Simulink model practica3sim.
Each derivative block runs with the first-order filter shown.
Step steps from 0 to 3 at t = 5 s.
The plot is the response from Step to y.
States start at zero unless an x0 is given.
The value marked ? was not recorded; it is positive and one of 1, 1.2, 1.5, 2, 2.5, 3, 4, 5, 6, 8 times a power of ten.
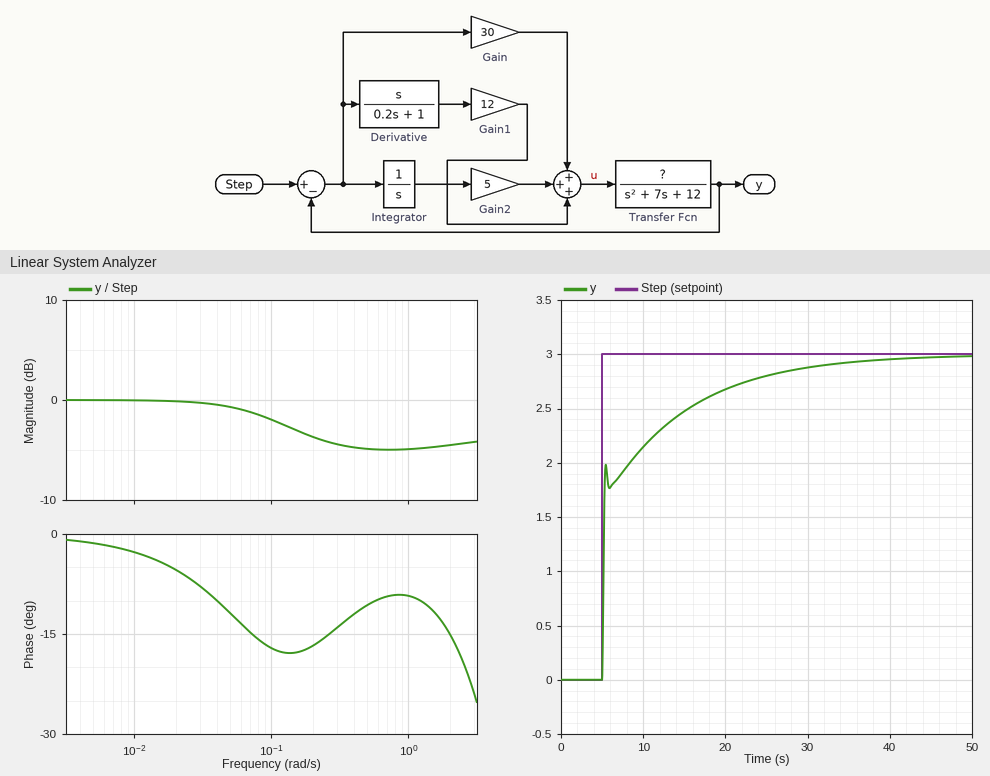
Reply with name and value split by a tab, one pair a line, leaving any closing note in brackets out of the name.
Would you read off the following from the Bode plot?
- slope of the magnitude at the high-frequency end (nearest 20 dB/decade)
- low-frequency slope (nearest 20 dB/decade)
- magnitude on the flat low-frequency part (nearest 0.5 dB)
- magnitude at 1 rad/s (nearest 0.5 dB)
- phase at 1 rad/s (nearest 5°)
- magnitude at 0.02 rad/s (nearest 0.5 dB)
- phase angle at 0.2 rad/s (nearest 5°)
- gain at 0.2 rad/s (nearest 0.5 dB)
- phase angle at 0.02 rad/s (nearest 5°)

slope of the magnitude at the high-frequency end	0 dB/decade
low-frequency slope	0 dB/decade
magnitude on the flat low-frequency part	0.0 dB
magnitude at 1 rad/s	-5.0 dB
phase at 1 rad/s	-10°
magnitude at 0.02 rad/s	0.0 dB
phase angle at 0.2 rad/s	-15°
gain at 0.2 rad/s	-3.5 dB
phase angle at 0.02 rad/s	-5°
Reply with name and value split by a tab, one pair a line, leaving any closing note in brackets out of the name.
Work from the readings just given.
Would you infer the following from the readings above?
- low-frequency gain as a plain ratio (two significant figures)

low-frequency gain as a plain ratio	1.0
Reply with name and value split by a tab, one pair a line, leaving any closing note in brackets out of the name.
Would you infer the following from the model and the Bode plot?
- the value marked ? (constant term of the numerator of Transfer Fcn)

the value marked ?	0.5
